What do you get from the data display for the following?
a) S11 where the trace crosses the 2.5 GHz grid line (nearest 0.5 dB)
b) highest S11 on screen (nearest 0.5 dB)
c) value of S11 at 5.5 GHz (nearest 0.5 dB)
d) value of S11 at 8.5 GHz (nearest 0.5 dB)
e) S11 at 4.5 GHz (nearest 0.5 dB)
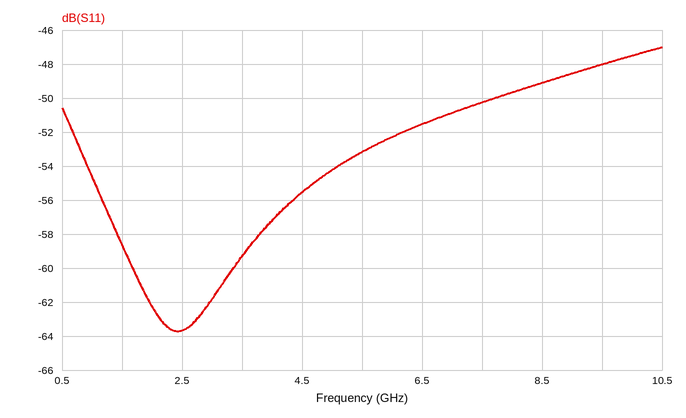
-63.5 dB
-47.0 dB
-53.0 dB
-49.0 dB
-55.5 dB
